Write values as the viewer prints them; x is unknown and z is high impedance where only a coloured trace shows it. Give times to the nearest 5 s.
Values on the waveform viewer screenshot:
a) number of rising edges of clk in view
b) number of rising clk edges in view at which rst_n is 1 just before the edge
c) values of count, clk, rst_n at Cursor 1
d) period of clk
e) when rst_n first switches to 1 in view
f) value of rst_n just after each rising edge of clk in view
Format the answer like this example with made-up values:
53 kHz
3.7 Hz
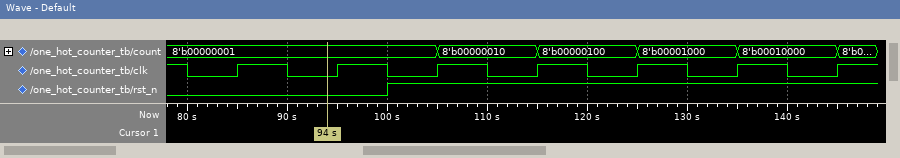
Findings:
7
5
count=8'b00000001, clk=0, rst_n=0
10 s
100 s
0 0 1 1 1 1 1
